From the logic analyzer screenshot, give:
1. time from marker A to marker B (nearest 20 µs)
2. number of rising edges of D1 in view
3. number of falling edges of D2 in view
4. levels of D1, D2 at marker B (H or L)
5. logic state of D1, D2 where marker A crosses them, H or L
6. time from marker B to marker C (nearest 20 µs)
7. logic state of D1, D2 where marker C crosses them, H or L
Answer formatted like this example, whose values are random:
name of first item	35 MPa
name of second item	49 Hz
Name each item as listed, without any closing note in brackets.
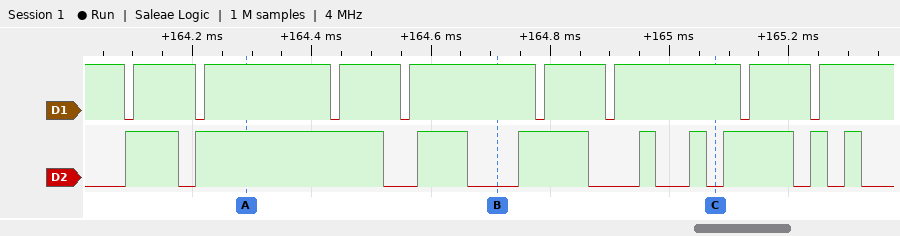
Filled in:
time from marker A to marker B	420 µs
number of rising edges of D1 in view	8
number of falling edges of D2 in view	9
levels of D1, D2 at marker B	D1=H, D2=L
logic state of D1, D2 where marker A crosses them, H or L	D1=H, D2=H
time from marker B to marker C	360 µs
logic state of D1, D2 where marker C crosses them, H or L	D1=H, D2=L
